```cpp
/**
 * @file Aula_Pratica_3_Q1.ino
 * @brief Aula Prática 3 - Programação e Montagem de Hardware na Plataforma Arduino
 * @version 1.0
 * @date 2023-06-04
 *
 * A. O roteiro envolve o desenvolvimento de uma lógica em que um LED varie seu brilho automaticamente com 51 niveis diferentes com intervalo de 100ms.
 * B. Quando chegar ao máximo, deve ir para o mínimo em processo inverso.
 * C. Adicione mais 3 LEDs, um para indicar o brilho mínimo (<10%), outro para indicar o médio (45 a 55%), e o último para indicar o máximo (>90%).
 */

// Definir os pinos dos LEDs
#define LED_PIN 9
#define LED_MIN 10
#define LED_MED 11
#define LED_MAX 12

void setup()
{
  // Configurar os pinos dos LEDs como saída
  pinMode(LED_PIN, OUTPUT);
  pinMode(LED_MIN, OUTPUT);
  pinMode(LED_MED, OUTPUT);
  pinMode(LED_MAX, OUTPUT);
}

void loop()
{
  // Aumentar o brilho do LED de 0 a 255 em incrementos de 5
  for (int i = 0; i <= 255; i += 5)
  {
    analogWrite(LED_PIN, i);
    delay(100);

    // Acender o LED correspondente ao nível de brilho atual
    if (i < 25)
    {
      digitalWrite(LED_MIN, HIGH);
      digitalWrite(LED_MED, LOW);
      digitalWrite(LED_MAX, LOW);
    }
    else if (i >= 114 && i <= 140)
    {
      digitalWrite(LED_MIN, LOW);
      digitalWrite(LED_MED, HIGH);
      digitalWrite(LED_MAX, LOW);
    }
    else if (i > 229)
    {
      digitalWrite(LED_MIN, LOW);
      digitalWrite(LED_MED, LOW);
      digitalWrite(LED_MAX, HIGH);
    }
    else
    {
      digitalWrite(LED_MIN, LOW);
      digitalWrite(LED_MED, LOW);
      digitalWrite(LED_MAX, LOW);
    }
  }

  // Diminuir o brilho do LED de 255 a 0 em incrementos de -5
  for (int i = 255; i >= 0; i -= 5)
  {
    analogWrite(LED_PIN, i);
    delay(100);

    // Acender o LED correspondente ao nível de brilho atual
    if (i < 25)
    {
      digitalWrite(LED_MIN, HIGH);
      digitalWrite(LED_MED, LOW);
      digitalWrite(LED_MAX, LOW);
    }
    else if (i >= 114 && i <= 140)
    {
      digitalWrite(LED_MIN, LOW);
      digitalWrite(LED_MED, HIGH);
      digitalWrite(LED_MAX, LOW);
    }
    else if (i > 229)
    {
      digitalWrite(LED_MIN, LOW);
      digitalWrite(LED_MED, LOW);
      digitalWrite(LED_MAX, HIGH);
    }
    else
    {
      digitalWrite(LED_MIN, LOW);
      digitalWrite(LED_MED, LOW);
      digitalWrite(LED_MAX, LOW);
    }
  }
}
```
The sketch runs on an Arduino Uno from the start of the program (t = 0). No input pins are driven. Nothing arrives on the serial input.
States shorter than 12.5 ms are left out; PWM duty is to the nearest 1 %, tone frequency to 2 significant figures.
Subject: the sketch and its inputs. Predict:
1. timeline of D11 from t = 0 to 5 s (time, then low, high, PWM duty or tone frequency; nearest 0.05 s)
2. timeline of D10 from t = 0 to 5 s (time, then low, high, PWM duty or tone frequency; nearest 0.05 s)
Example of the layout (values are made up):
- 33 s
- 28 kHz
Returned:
- 0 s low; 2.4 s high; 3 s low
- 0 s low; 0.1 s high; 0.6 s low
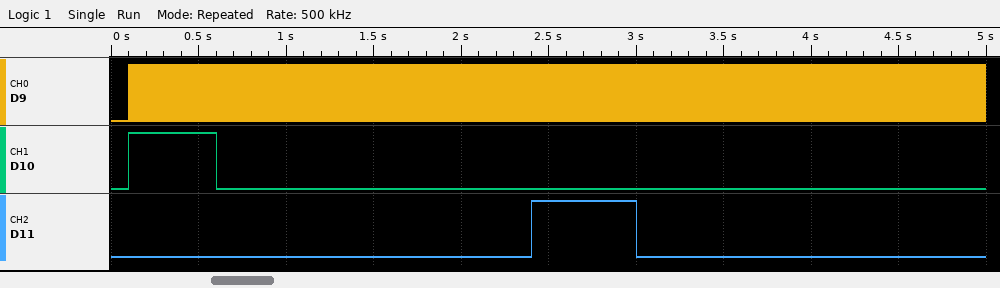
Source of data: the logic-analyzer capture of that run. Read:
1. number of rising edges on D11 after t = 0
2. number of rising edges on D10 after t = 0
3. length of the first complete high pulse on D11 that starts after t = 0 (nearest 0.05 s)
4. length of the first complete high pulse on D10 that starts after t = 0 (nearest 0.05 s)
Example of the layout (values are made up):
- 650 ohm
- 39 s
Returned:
- 1
- 1
- 0.60 s
- 0.50 s
